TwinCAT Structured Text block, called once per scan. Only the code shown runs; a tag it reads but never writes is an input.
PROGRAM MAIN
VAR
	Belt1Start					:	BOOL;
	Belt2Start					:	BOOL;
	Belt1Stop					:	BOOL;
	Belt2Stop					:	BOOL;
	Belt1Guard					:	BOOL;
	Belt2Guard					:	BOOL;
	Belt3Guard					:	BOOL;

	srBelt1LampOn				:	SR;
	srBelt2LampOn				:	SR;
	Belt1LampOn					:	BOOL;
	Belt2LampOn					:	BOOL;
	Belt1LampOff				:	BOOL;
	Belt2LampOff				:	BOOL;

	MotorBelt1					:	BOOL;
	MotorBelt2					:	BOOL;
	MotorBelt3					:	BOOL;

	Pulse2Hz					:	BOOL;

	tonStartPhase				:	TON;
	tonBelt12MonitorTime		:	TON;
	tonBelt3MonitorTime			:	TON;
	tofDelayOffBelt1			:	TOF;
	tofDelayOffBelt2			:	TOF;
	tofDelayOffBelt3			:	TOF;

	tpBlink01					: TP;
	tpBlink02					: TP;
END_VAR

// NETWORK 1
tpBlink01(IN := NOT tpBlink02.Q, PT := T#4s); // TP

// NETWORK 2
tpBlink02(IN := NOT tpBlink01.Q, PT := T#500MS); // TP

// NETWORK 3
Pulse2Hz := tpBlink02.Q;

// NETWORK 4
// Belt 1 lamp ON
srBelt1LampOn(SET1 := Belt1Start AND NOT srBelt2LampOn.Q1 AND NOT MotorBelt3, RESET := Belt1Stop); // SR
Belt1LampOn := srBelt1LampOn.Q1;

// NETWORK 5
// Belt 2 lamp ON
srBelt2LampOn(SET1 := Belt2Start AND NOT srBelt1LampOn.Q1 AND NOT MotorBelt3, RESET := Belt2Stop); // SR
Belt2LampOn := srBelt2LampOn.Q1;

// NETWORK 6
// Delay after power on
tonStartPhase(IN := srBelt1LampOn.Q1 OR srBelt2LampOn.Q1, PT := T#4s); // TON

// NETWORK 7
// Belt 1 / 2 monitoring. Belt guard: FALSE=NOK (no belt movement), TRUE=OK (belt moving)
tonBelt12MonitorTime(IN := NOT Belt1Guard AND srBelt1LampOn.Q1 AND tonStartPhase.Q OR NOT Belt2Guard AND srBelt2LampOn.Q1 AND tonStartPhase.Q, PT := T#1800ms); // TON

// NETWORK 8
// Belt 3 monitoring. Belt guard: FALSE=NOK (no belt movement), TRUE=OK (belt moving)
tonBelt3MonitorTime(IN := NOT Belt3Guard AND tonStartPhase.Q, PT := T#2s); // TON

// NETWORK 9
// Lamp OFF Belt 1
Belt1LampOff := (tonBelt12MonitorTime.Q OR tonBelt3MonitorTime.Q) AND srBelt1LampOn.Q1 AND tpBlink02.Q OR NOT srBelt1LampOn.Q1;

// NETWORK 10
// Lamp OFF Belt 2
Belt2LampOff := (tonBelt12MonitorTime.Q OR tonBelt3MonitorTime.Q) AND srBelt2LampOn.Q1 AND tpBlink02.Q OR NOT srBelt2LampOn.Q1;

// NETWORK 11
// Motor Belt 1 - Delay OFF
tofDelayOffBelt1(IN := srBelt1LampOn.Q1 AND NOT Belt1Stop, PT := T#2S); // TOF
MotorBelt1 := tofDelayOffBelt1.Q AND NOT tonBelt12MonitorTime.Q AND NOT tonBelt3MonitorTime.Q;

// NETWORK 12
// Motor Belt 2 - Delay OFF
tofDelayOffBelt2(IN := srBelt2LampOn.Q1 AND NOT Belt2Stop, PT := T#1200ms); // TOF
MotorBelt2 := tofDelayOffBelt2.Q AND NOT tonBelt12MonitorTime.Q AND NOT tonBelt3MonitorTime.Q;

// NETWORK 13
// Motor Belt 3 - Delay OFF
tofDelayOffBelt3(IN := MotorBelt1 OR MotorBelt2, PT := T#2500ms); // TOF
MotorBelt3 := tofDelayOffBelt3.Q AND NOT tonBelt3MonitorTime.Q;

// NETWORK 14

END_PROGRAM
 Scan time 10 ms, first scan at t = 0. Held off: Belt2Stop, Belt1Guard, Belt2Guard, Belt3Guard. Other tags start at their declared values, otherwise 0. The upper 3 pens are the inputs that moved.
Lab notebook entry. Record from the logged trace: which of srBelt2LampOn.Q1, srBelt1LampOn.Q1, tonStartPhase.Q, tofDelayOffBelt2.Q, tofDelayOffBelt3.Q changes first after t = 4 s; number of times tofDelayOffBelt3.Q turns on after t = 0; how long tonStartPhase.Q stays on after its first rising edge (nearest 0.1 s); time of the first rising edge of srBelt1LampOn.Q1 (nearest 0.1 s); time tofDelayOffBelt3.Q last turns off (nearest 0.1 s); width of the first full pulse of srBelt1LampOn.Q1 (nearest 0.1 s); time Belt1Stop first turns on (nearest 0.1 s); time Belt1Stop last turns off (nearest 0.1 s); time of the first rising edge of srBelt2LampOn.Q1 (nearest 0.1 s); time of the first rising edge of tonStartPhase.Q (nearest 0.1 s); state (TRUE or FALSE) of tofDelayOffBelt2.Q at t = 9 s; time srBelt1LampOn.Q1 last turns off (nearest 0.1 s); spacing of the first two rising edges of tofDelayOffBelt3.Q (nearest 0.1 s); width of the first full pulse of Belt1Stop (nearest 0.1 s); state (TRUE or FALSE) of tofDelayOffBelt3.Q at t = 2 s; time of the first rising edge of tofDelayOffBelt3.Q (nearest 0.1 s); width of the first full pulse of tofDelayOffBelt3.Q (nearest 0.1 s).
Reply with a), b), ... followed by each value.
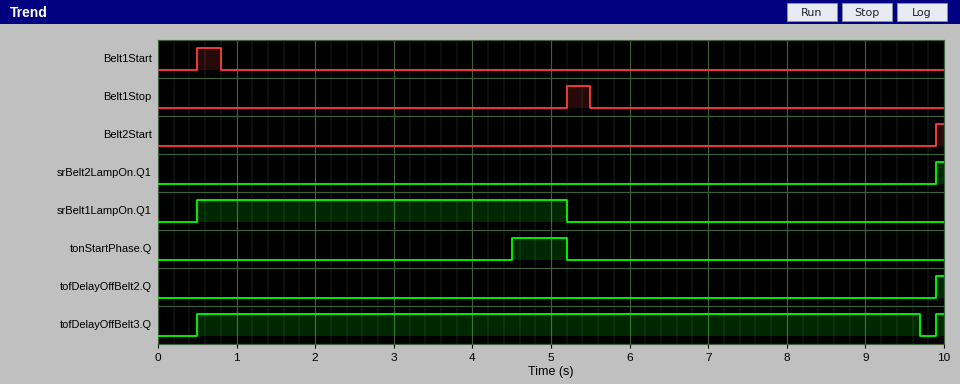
a) tonStartPhase.Q
b) 2
c) 0.7 s
d) 0.5 s
e) 9.7 s
f) 4.7 s
g) 5.2 s
h) 5.5 s
i) 9.9 s
j) 4.5 s
k) FALSE
l) 5.2 s
m) 9.4 s
n) 0.3 s
o) TRUE
p) 0.5 s
q) 9.2 s
